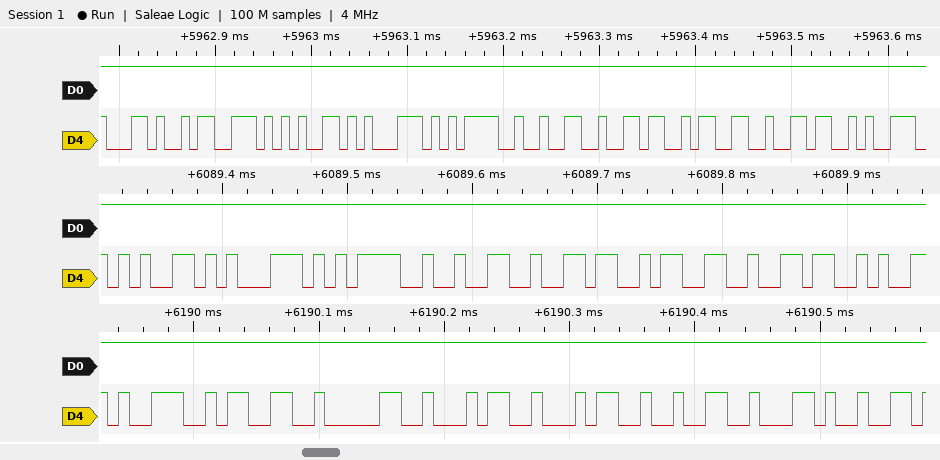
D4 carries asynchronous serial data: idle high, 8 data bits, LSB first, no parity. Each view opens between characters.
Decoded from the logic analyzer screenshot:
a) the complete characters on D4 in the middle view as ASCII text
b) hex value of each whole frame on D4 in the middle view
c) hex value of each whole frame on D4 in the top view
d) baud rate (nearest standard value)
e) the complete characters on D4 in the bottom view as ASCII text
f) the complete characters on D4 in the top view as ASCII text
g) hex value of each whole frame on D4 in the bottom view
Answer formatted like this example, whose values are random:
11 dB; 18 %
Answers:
"eq=2636"; 65, 71, 3D, 32, 36, 33, 36; 2C, 73, 65, 71, 3D, 32, 36, 33, 36; 115200 baud; "930442,"; ",seq=2636"; 39, 33, 30, 34, 34, 32, 2C
